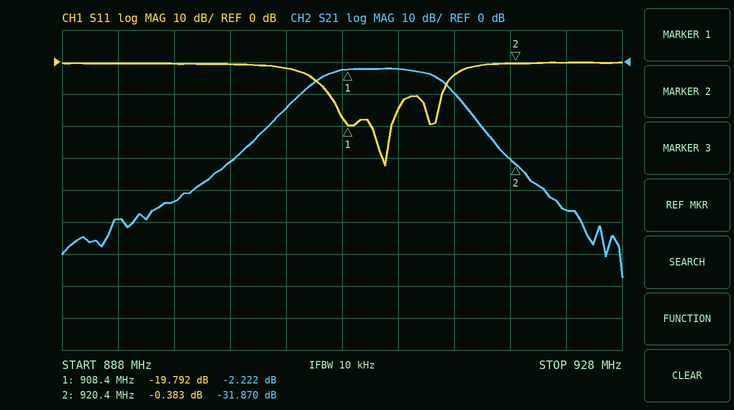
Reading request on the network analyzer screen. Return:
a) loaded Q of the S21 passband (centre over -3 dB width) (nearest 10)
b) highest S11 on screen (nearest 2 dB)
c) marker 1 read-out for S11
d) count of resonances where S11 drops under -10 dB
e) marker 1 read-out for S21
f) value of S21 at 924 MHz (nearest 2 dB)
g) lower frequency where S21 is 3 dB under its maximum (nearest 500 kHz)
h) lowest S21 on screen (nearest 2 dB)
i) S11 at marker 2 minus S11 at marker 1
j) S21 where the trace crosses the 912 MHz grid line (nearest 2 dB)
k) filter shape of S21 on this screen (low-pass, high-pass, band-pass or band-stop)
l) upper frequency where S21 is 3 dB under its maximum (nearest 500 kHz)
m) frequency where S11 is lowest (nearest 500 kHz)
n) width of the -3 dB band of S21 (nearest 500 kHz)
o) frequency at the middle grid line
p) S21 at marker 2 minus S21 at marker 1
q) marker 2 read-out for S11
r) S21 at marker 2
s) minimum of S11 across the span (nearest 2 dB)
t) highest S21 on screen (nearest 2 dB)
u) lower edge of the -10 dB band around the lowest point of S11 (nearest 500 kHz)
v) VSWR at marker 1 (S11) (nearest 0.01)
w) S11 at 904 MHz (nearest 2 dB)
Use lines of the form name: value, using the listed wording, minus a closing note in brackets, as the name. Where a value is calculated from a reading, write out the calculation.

loaded Q of the S21 passband (centre over -3 dB width): 910.75 MHz / 8.5 MHz ≈ 107, so 110 to the nearest 10
highest S11 on screen: 0 dB
marker 1 read-out for S11: -19.792 dB
count of resonances where S11 drops under -10 dB: 2
marker 1 read-out for S21: -2.222 dB
value of S21 at 924 MHz: -46 dB
lower frequency where S21 is 3 dB under its maximum: 906.5 MHz
lowest S21 on screen: -68 dB
S11 at marker 2 minus S11 at marker 1: -0.383 − (-19.792) = 19.409 dB
S21 where the trace crosses the 912 MHz grid line: -2 dB
filter shape of S21 on this screen: band-pass
upper frequency where S21 is 3 dB under its maximum: 915.0 MHz
frequency where S11 is lowest: 911.0 MHz
width of the -3 dB band of S21: 915.0 MHz − 906.5 MHz = 8.5 MHz
frequency at the middle grid line: 908 MHz
S21 at marker 2 minus S21 at marker 1: -31.87 − (-2.222) = -29.648 dB
marker 2 read-out for S11: -0.383 dB
S21 at marker 2: -31.870 dB
minimum of S11 across the span: -32 dB
highest S21 on screen: -2 dB
lower edge of the -10 dB band around the lowest point of S11: 907.0 MHz
VSWR at marker 1 (S11): (1 + 0.1024)/(1 − 0.1024) ≈ 1.23
S11 at 904 MHz: -2 dB
